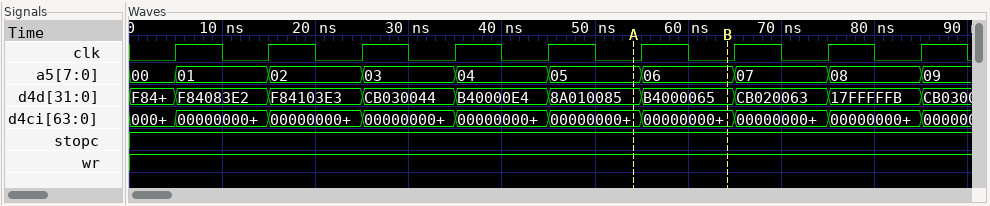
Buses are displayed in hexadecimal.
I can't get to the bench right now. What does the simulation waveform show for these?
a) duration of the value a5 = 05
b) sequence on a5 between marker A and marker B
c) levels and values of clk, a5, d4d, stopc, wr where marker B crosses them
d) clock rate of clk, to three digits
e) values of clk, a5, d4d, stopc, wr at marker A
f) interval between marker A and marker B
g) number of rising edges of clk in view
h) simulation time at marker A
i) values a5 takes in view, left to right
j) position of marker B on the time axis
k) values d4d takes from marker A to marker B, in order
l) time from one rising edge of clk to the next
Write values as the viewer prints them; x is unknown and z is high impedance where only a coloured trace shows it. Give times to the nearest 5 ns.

10 ns
05, 06
clk=0, a5=06, d4d=B4000065, stopc=1, wr=1
100 MHz
clk=0, a5=05, d4d=8A010085, stopc=1, wr=1
10 ns
9
55 ns
00, 01, 02, 03, 04, 05, 06, 07, 08, 09
65 ns
8A010085, B4000065
10 ns
